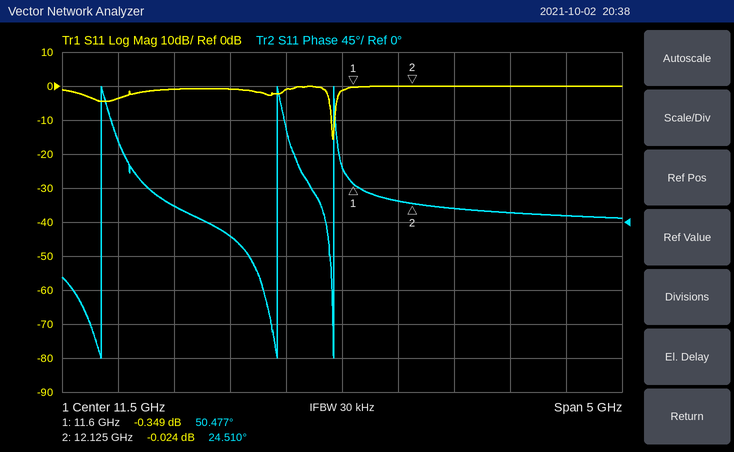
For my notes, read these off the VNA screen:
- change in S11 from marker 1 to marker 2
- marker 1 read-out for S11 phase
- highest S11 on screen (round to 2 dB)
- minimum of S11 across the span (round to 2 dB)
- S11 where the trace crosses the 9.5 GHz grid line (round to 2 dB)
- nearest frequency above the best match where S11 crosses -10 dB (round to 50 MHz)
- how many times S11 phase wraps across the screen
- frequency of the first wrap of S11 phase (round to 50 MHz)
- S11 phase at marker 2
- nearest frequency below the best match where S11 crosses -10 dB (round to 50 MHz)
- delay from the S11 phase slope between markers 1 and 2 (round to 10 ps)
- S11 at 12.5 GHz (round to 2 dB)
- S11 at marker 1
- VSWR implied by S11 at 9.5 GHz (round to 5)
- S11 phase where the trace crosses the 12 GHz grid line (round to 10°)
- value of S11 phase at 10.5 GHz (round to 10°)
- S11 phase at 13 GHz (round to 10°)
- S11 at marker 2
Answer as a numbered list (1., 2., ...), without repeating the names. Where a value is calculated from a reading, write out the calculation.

1. -0.024 − (-0.349) = 0.325 dB
2. 50.477°
3. 0 dB
4. -16 dB
5. -4 dB
6. 11.45 GHz
7. 3
8. 9.35 GHz
9. 24.510°
10. 11.40 GHz
11. −(24.51° − (50.477°))/(360° × 525 MHz) ≈ 137 ps, so 140 ps to the nearest 10 ps
12. 0 dB
13. -0.349 dB
14. |Γ| = 10^(-4/20) = 0.6310; VSWR = (1 + 0.6310)/(1 − 0.6310) ≈ 4.42, so 5 to the nearest 5
15. 30°
16. -20°
17. 10°
18. -0.024 dB
